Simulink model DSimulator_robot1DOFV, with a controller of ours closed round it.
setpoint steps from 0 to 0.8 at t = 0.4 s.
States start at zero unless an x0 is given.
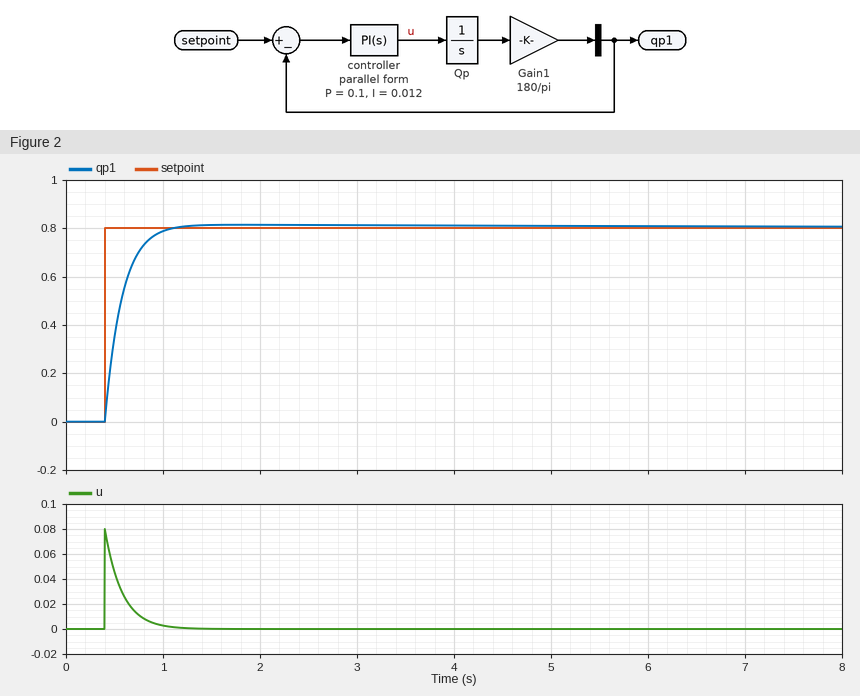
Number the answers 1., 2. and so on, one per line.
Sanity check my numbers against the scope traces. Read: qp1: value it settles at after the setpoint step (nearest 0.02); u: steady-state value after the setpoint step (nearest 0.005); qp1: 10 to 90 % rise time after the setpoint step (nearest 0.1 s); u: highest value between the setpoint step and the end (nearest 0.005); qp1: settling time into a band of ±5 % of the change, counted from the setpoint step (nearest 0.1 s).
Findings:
1. 0.80
2. 0.000
3. 0.4 s
4. 0.080
5. 0.5 s
